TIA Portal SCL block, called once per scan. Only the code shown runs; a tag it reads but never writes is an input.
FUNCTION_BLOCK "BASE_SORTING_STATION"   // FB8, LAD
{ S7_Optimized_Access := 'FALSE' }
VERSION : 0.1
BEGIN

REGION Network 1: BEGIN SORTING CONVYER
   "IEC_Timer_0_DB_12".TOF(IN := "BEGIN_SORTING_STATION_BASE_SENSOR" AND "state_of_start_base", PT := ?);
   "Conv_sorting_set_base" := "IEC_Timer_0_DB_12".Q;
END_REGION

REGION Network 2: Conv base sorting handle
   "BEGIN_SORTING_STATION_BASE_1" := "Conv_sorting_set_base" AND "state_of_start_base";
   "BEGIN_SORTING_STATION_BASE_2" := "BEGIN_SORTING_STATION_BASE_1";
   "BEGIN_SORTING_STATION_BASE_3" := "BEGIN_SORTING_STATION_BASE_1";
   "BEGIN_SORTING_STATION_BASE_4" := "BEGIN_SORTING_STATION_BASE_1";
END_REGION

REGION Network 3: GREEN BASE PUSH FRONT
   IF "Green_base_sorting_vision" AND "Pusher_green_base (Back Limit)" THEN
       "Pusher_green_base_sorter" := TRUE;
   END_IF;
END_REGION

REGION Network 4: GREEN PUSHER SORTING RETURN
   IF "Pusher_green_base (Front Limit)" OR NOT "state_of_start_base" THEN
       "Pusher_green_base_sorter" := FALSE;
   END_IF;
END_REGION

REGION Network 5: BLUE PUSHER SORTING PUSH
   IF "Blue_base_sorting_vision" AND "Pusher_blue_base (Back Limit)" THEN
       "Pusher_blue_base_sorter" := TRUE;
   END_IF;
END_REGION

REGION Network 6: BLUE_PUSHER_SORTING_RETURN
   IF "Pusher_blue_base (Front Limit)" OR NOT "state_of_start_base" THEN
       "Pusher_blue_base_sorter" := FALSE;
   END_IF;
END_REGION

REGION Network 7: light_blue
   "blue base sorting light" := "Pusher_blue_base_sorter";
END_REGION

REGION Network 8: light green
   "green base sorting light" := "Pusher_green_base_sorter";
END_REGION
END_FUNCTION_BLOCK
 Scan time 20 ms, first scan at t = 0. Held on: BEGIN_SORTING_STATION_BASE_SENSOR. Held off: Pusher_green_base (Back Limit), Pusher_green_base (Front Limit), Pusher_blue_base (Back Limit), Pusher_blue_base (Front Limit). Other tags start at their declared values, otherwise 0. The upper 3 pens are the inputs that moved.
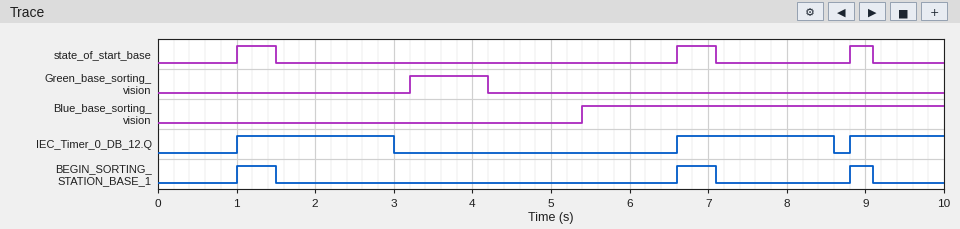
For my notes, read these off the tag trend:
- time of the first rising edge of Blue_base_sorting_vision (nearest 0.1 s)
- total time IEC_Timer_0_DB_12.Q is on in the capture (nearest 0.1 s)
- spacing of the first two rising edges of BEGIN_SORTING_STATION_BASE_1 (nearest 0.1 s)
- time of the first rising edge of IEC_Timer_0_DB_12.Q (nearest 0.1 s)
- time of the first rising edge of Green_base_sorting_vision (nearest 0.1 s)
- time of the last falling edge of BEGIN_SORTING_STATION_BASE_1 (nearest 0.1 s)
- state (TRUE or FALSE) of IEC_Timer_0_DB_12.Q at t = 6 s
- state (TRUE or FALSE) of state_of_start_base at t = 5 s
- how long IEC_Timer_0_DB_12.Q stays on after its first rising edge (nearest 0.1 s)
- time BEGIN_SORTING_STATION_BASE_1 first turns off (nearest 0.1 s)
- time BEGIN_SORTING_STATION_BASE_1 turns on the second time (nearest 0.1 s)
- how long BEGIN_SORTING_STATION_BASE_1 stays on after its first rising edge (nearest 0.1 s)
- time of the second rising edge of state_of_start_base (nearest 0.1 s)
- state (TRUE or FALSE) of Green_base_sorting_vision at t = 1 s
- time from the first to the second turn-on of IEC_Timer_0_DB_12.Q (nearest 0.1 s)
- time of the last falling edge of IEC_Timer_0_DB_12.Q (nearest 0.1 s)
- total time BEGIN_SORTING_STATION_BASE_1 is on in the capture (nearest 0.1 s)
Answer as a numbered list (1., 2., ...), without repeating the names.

1. 5.4 s
2. 5.2 s
3. 5.6 s
4. 1.0 s
5. 3.2 s
6. 9.1 s
7. FALSE
8. FALSE
9. 2.0 s
10. 1.5 s
11. 6.6 s
12. 0.5 s
13. 6.6 s
14. FALSE
15. 5.6 s
16. 8.6 s
17. 1.3 s
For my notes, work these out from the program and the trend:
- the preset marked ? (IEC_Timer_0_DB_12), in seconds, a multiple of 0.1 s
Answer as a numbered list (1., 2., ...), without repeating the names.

1. 1.5 s
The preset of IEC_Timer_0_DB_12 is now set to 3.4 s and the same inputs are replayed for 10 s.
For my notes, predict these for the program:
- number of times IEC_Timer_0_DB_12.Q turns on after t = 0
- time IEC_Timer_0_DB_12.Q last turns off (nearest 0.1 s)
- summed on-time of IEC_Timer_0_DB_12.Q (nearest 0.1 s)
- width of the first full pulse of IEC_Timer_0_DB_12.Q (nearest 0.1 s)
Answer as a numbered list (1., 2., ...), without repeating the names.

1. 2
2. 4.9 s
3. 7.3 s
4. 3.9 s
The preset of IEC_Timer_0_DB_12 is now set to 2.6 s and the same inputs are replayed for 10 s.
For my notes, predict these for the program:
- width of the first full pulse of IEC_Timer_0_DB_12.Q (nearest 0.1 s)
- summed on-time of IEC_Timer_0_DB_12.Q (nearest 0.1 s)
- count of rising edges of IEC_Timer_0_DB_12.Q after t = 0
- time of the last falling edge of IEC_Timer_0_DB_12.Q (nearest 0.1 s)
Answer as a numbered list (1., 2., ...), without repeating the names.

1. 3.1 s
2. 6.5 s
3. 2
4. 4.1 s
